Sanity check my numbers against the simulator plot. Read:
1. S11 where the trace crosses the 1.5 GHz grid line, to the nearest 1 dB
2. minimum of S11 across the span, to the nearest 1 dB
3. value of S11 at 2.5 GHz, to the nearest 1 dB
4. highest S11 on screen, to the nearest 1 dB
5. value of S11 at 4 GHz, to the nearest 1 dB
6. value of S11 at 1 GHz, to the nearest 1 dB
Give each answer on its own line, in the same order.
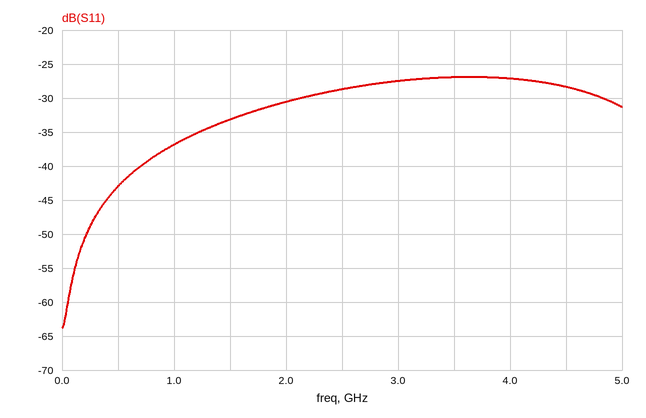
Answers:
-33 dB
-64 dB
-29 dB
-27 dB
-27 dB
-37 dB
